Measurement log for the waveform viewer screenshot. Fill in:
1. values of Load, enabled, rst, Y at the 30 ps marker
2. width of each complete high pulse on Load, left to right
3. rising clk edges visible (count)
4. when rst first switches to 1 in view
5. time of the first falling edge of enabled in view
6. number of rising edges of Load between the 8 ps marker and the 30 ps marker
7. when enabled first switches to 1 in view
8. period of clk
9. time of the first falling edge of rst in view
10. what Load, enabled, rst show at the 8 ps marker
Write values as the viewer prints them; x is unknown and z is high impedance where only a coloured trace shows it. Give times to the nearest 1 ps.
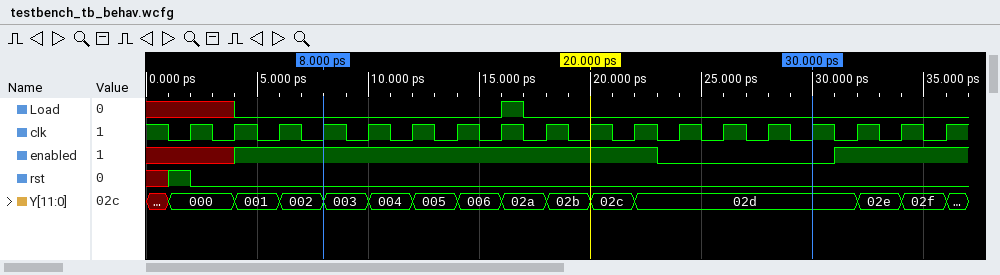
Load=0, enabled=0, rst=0, Y=02d
1 ps
18
1 ps
23 ps
1
4 ps
2 ps
2 ps
Load=0, enabled=1, rst=0
